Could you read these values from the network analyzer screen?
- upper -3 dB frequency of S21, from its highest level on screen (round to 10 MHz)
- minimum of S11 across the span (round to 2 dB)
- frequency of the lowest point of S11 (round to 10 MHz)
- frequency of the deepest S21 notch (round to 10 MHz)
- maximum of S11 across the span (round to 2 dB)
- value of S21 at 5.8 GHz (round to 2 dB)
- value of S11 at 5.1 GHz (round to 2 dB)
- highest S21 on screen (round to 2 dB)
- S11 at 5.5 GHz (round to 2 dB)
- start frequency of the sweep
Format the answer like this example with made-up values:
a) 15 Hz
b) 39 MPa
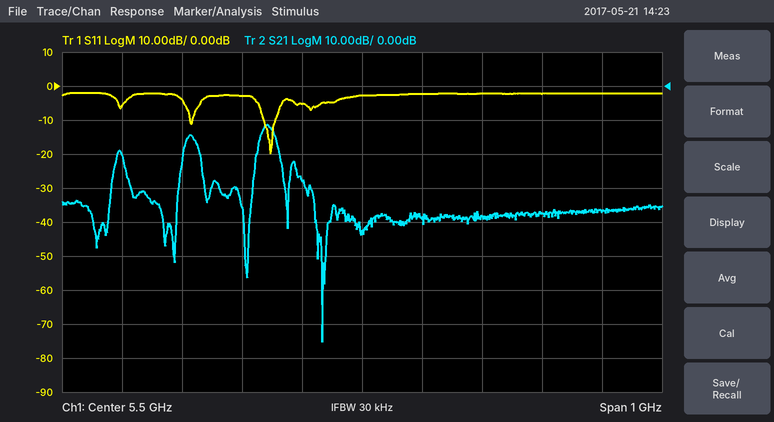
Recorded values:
a) 5.35 GHz
b) -20 dB
c) 5.35 GHz
d) 5.43 GHz
e) -2 dB
f) -38 dB
g) -6 dB
h) -12 dB
i) -2 dB
j) 5 GHz
